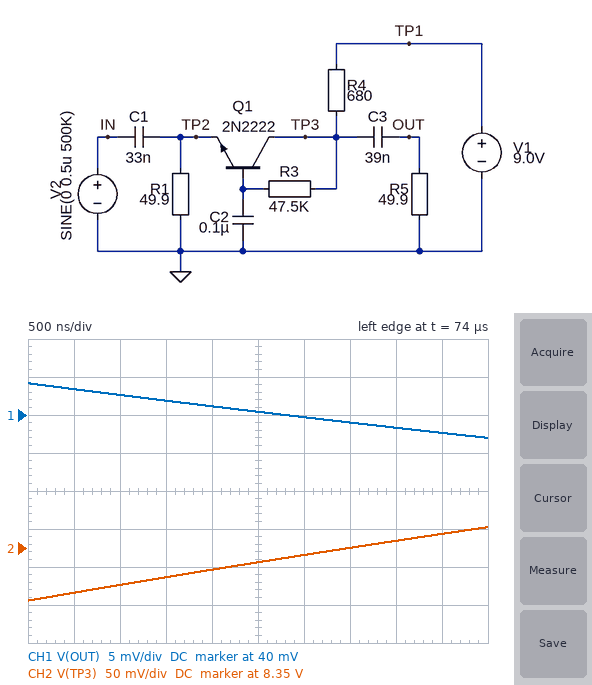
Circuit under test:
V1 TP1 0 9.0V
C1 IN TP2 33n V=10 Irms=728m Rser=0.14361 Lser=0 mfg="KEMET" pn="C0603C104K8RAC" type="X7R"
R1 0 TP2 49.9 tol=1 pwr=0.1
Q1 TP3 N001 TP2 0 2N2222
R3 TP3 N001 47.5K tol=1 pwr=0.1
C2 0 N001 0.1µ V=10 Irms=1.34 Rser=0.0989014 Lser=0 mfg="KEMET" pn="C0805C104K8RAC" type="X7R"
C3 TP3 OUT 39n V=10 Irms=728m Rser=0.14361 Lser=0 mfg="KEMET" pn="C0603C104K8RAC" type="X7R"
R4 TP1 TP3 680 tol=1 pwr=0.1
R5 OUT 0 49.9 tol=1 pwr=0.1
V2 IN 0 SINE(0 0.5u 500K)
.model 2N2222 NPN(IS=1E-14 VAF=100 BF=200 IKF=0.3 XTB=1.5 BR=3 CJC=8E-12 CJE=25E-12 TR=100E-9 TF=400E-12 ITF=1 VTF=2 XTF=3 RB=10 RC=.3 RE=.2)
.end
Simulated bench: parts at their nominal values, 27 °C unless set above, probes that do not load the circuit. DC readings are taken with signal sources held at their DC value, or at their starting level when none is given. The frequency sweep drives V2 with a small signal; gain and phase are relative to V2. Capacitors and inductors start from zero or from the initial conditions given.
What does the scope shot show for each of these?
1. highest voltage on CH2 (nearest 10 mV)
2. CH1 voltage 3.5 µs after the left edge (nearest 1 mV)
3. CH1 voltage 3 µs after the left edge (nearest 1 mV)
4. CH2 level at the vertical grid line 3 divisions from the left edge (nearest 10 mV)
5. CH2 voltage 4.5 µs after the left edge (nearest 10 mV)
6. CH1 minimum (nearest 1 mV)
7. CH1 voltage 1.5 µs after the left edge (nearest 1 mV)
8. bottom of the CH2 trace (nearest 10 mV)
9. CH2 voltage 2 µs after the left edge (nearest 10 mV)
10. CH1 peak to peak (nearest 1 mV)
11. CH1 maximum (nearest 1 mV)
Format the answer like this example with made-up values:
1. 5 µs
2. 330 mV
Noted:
1. 8.38 V
2. 39 mV
3. 40 mV
4. 8.31 V
5. 8.37 V
6. 37 mV
7. 42 mV
8. 8.28 V
9. 8.32 V
10. 7 mV
11. 44 mV
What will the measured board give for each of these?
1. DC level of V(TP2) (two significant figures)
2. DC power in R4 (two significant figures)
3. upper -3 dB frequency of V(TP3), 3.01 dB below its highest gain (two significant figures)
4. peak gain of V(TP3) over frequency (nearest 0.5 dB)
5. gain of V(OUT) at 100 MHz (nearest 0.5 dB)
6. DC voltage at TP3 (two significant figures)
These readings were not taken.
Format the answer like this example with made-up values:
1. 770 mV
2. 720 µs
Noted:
1. 430 mV
2. 50 mW
3. 68 MHz
4. 22.5 dB
5. 17.0 dB
6. 3.2 V
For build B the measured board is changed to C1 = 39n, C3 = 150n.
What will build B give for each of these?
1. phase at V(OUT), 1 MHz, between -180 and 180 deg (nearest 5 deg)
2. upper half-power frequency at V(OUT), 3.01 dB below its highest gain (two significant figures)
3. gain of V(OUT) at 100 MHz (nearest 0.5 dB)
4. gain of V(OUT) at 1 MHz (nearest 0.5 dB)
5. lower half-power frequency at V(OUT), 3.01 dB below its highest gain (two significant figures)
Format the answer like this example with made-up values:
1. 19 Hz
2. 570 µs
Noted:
1. 50 deg
2. 67 MHz
3. 17.0 dB
4. 18.5 dB
5. 1.2 MHz
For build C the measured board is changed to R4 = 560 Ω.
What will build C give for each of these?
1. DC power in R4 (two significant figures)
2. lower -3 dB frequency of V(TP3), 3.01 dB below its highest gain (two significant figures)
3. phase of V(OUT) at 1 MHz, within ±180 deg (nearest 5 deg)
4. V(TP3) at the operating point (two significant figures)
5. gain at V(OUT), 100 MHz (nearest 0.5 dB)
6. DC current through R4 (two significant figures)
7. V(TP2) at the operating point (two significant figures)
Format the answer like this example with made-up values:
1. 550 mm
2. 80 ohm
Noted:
1. 53 mW
2. 1.6 MHz
3. 60 deg
4. 3.5 V
5. 17.5 dB
6. 9.8 mA
7. 490 mV
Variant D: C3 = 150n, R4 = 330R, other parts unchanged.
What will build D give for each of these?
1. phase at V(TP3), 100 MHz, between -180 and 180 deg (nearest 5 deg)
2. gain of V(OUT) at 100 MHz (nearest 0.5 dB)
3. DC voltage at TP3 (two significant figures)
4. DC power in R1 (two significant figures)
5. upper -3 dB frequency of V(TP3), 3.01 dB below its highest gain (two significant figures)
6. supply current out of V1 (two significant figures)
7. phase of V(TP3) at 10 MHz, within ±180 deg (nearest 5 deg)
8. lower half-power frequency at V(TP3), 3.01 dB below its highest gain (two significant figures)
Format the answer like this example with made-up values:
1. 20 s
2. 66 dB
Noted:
1. -65 deg
2. 18.5 dB
3. 4.6 V
4. 8.9 mW
5. 55 MHz
6. 13 mA
7. 0 deg
8. 2.0 MHz
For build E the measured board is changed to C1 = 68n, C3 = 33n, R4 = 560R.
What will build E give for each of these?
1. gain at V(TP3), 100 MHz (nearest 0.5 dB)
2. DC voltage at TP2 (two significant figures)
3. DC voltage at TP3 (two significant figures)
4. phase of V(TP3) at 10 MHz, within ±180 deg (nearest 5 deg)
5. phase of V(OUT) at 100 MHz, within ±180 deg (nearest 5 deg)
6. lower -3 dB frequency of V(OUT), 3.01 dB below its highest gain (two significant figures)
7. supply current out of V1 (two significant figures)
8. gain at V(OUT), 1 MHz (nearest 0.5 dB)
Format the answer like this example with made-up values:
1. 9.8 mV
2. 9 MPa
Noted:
1. 17.5 dB
2. 490 mV
3. 3.5 V
4. -5 deg
5. -60 deg
6. 780 kHz
7. 9.8 mA
8. 21.0 dB
